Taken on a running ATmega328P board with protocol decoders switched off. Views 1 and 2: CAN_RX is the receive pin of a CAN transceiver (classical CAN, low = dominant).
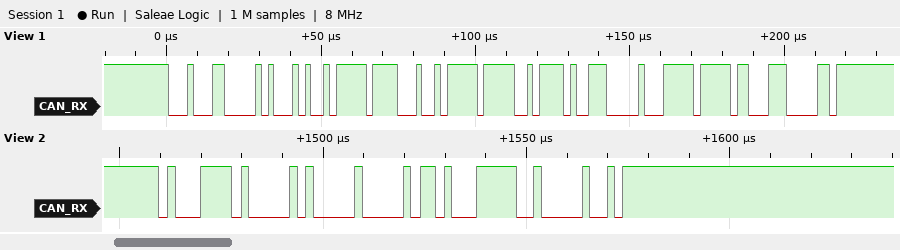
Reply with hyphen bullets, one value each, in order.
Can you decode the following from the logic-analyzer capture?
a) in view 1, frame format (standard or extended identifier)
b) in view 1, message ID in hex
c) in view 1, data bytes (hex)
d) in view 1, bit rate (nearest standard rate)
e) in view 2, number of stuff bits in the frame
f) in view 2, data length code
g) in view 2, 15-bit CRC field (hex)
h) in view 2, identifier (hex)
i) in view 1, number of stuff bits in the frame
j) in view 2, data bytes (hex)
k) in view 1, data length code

- standard
- 0x118
- A5 FF 12 FF D7 A7 00 FF
- 500 kbit/s
- 5
- 2
- 0x3E80
- 0x47A
- 8
- 00 34
- 8
